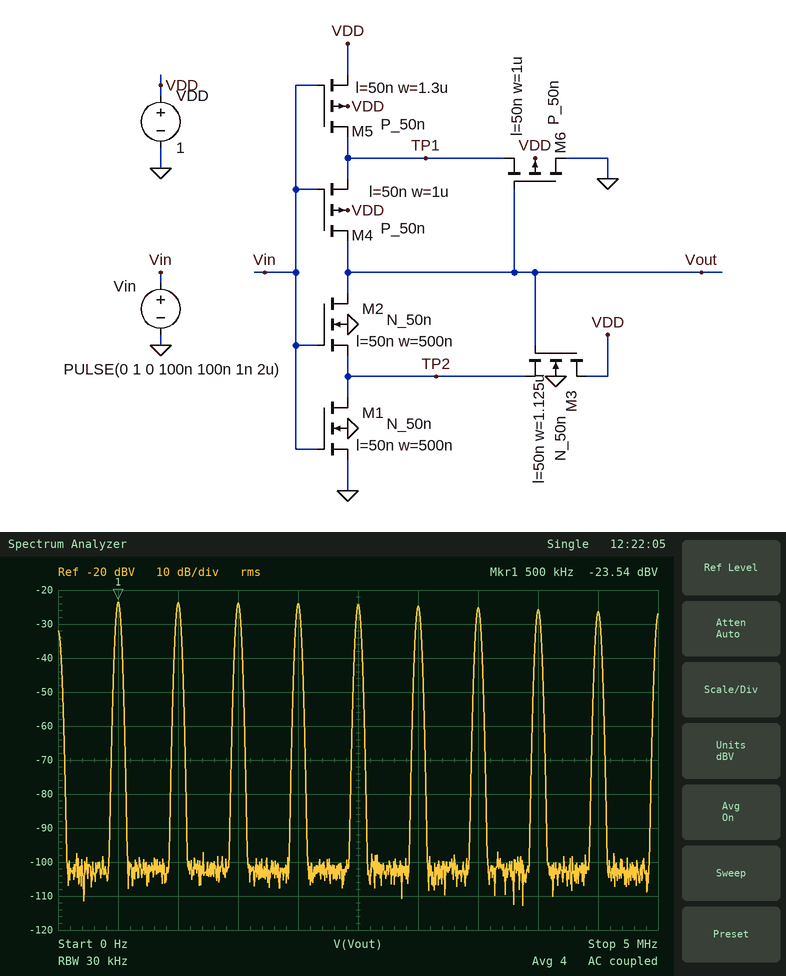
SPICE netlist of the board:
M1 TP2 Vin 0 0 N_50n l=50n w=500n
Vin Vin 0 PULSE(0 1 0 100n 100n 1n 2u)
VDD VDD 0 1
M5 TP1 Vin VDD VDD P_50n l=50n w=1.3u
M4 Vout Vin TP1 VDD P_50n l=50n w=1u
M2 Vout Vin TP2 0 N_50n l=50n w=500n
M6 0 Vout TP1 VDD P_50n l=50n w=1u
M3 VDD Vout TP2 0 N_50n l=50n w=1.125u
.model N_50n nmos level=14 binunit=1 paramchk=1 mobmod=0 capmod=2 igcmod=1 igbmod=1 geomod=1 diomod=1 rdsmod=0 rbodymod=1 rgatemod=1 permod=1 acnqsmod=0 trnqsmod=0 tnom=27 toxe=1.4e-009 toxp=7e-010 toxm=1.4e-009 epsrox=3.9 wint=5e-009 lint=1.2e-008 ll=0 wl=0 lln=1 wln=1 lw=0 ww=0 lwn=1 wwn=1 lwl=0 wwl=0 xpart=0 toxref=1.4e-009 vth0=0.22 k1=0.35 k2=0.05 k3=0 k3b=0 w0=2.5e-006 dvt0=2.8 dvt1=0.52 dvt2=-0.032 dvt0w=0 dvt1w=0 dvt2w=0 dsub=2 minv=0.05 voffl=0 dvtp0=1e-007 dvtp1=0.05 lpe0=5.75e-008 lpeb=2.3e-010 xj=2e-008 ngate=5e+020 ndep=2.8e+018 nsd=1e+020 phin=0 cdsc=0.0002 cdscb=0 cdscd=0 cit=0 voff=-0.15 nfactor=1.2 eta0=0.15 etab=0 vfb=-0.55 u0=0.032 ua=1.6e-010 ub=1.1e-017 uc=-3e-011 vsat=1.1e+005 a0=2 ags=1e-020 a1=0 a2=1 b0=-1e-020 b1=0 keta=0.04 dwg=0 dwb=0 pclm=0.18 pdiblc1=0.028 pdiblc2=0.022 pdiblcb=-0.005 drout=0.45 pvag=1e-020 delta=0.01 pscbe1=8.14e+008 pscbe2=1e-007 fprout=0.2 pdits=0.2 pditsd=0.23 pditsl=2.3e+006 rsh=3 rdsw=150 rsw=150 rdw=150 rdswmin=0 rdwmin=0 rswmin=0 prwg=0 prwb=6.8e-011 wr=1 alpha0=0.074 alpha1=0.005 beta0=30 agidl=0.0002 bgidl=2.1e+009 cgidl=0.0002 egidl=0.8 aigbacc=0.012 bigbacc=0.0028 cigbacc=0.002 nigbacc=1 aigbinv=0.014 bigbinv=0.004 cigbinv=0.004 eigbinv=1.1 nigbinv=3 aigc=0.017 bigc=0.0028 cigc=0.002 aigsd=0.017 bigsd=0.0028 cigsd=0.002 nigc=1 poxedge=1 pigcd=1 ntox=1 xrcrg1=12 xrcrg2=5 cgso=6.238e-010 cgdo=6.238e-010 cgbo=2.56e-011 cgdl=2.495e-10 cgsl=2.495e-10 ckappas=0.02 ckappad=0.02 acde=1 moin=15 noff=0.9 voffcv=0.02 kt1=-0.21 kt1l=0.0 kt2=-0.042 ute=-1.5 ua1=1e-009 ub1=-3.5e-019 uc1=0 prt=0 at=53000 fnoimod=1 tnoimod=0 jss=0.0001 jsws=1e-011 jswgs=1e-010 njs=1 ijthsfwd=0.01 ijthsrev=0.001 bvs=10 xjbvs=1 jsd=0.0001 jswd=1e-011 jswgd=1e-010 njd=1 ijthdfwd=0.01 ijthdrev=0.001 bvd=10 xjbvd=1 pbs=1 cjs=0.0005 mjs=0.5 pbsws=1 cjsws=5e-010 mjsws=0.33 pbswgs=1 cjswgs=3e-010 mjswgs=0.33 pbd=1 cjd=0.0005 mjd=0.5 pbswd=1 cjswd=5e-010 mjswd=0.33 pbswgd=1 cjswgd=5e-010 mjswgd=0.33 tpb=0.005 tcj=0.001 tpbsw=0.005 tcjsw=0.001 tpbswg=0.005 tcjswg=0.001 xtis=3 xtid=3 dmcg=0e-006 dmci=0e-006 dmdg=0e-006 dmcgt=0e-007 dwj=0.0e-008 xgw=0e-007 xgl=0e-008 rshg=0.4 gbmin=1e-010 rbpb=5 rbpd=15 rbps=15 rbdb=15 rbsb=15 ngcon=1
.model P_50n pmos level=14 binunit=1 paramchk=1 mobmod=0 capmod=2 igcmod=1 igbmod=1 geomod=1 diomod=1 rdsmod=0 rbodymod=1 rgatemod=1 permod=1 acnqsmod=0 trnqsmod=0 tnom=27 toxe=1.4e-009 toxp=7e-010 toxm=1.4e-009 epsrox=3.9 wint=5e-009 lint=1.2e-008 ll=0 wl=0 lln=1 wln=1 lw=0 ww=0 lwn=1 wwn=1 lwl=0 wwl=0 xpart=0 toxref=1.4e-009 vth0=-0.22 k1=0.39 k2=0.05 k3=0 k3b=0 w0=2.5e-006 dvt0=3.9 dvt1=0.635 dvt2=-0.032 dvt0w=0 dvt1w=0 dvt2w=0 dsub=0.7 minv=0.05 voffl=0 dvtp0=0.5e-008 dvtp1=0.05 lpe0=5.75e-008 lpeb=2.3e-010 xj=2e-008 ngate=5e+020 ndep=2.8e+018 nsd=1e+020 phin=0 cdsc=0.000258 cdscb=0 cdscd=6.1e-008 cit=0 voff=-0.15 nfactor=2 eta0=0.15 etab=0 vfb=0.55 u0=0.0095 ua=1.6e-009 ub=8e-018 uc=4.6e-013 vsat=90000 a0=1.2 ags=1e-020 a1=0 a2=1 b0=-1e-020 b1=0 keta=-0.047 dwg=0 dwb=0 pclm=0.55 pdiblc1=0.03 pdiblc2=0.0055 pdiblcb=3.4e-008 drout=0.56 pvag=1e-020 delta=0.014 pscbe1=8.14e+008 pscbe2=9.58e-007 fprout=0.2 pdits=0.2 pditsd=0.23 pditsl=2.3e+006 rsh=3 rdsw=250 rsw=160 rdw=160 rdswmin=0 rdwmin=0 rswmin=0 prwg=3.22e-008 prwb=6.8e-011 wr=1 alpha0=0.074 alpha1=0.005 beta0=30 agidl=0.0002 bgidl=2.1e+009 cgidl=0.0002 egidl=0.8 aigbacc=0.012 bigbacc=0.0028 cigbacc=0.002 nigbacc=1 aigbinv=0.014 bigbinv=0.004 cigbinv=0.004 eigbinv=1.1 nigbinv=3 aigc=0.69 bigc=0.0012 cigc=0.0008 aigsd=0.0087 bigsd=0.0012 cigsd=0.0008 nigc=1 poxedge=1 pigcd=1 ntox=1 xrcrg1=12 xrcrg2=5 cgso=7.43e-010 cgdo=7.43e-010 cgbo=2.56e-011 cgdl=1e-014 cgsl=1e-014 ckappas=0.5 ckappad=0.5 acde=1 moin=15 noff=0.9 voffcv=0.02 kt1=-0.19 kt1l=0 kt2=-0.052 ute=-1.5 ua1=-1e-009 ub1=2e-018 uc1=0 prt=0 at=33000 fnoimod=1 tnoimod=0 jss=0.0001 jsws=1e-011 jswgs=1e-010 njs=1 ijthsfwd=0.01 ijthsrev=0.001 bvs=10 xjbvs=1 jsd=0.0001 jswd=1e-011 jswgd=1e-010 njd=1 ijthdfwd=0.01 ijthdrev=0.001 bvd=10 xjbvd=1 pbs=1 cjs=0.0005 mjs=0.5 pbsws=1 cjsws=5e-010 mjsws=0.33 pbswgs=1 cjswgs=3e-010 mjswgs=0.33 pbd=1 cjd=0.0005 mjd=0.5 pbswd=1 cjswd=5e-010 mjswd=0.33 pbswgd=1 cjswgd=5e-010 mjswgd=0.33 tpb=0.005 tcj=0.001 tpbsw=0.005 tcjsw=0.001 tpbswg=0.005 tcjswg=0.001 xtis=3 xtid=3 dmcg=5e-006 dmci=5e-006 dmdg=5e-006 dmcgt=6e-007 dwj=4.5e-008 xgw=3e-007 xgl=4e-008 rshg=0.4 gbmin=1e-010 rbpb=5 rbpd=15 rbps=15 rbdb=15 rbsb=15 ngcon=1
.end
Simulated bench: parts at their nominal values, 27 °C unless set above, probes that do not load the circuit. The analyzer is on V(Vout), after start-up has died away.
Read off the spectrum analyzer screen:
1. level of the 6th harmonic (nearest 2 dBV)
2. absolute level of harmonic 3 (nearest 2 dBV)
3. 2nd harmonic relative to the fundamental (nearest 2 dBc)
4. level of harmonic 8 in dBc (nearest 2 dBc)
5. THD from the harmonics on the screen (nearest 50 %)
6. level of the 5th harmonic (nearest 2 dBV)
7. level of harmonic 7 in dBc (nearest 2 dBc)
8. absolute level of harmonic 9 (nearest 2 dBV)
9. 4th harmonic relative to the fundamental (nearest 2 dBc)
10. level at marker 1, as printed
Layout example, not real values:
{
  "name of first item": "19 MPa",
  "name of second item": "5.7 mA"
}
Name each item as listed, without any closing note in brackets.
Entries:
{
  "level of the 6th harmonic": "-24 dBV",
  "absolute level of harmonic 3": "-24 dBV",
  "2nd harmonic relative to the fundamental": "0 dBc",
  "level of harmonic 8 in dBc": "-2 dBc",
  "THD from the harmonics on the screen": "250 %",
  "level of the 5th harmonic": "-24 dBV",
  "level of harmonic 7 in dBc": "-2 dBc",
  "absolute level of harmonic 9": "-26 dBV",
  "4th harmonic relative to the fundamental": "0 dBc",
  "level at marker 1, as printed": "-23.54 dBV"
}
